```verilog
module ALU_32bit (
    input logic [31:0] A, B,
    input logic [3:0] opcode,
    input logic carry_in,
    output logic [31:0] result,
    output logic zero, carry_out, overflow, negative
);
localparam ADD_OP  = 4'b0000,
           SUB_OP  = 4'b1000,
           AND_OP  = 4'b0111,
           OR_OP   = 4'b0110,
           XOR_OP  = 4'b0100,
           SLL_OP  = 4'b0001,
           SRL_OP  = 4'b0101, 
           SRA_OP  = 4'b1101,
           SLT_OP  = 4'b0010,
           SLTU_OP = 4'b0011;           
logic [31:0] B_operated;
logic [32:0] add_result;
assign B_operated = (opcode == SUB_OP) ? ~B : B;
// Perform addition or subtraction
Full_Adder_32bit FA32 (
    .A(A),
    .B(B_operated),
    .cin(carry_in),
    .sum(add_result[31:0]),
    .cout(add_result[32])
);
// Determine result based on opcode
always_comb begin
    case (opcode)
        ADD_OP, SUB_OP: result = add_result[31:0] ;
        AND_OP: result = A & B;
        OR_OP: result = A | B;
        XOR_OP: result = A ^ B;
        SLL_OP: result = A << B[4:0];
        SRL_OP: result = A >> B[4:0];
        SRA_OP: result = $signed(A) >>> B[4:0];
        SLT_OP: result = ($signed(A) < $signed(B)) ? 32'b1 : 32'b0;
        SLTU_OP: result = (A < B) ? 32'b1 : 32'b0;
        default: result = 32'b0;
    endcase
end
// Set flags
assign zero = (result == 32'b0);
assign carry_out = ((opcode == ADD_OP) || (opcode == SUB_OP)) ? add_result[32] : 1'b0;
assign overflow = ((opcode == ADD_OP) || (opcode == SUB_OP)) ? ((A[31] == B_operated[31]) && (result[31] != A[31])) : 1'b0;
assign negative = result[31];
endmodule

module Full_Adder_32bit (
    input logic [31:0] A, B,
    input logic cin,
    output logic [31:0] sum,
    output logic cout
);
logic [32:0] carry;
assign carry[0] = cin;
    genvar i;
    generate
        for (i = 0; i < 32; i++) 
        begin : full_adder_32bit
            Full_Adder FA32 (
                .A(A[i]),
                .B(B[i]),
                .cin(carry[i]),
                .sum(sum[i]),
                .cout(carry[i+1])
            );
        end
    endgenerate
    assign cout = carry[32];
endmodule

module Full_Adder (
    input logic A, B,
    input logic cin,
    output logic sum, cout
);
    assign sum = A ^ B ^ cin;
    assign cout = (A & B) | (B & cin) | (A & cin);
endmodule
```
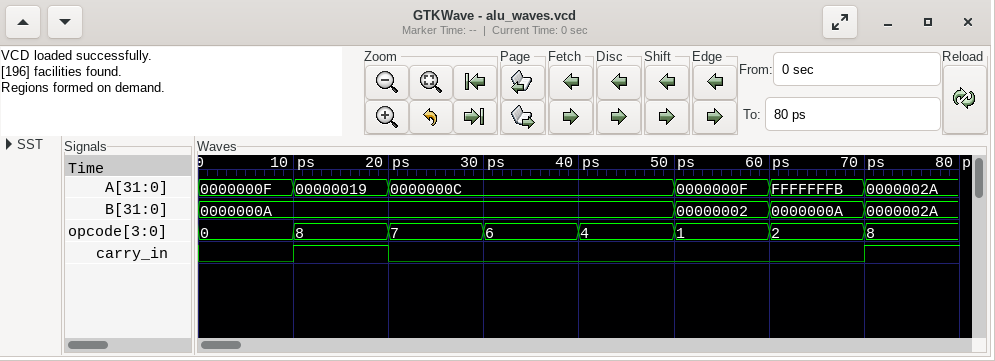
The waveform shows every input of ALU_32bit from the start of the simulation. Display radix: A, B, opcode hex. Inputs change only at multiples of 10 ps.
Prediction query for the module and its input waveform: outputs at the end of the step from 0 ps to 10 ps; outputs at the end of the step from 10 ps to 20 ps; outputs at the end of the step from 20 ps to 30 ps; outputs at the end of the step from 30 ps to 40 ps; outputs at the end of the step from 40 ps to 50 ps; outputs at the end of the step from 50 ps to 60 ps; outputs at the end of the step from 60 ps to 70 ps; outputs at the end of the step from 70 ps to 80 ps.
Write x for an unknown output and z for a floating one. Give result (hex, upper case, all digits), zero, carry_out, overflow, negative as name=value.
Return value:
result=00000019, zero=0, carry_out=0, overflow=0, negative=0
result=0000000F, zero=0, carry_out=1, overflow=0, negative=0
result=00000008, zero=0, carry_out=0, overflow=0, negative=0
result=0000000E, zero=0, carry_out=0, overflow=0, negative=0
result=00000006, zero=0, carry_out=0, overflow=0, negative=0
result=0000003C, zero=0, carry_out=0, overflow=0, negative=0
result=00000001, zero=0, carry_out=0, overflow=0, negative=0
result=00000000, zero=1, carry_out=1, overflow=0, negative=0
